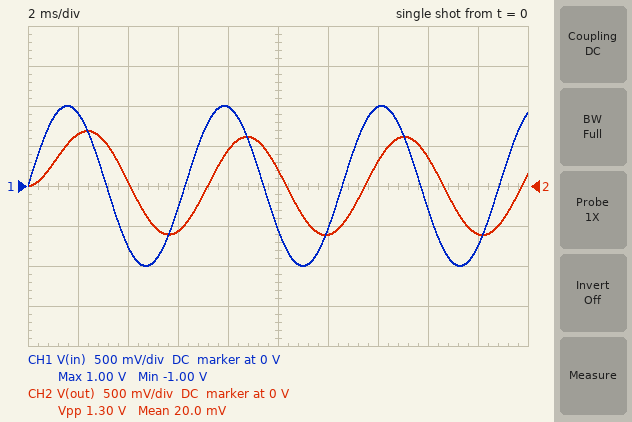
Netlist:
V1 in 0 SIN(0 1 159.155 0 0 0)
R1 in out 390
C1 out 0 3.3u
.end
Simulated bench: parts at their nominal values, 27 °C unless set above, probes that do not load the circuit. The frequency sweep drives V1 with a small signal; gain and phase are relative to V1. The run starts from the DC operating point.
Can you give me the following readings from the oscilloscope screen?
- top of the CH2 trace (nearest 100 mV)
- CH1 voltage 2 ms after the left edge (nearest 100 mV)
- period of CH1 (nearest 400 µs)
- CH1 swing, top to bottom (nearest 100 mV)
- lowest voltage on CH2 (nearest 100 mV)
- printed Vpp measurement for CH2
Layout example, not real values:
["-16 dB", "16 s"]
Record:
["700 mV", "900 mV", "6.4 ms", "2.0 V", "-600 mV", "1.30 V"]
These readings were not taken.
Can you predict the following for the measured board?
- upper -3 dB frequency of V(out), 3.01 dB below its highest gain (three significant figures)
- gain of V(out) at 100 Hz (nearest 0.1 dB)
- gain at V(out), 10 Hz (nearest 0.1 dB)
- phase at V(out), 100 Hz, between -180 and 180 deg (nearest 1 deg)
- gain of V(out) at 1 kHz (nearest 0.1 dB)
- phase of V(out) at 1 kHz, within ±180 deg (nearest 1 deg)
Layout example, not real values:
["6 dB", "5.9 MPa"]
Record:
["124 Hz", "-2.2 dB", "0 dB", "-39 deg", "-18.2 dB", "-83 deg"]
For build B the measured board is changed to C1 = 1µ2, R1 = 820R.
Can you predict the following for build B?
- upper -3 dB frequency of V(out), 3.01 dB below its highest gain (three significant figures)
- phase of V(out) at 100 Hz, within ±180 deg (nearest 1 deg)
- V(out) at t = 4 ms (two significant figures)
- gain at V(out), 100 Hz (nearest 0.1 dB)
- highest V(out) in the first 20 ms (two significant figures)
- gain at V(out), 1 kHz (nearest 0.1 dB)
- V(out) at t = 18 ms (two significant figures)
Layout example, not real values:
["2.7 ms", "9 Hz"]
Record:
["162 Hz", "-32 deg", "-49 mV", "-1.4 dB", "760 mV", "-15.9 dB", "-710 mV"]
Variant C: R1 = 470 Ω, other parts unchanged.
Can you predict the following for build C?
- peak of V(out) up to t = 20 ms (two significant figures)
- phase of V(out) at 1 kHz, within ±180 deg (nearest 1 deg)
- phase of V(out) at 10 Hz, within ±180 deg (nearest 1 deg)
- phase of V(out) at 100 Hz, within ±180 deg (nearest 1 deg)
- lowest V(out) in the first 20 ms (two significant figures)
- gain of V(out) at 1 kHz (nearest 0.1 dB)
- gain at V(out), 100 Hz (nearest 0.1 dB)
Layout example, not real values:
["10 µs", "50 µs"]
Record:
["630 mV", "-84 deg", "-6 deg", "-44 deg", "-540 mV", "-19.8 dB", "-2.9 dB"]
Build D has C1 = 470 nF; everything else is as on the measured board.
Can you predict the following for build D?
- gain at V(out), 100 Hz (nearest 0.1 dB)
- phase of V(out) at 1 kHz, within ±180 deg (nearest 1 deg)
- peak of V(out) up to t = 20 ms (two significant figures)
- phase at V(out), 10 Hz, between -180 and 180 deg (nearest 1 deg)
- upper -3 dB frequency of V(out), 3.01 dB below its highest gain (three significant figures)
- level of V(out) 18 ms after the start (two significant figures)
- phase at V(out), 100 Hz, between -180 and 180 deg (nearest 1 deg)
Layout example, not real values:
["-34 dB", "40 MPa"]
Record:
["-0.1 dB", "-49 deg", "980 mV", "-1 deg", "868 Hz", "-840 mV", "-7 deg"]
